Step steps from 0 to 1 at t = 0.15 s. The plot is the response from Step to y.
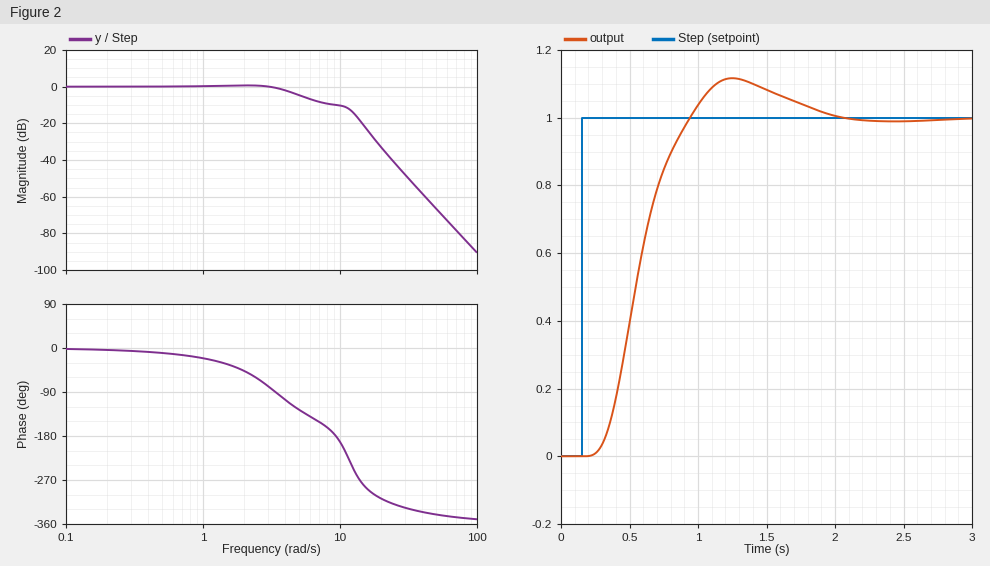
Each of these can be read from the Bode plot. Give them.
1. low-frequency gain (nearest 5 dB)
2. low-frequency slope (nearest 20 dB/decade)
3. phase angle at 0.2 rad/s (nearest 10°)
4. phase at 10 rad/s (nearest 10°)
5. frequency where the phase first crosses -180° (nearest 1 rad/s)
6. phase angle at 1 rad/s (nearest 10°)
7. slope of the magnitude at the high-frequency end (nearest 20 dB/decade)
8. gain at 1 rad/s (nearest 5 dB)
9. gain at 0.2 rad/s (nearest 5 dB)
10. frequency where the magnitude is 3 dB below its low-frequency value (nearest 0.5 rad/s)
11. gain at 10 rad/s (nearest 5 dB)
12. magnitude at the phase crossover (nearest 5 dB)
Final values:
0 dB
0 dB/decade
0°
-190°
9 rad/s
-20°
-80 dB/decade
0 dB
0 dB
4.5 rad/s
-10 dB
-10 dB
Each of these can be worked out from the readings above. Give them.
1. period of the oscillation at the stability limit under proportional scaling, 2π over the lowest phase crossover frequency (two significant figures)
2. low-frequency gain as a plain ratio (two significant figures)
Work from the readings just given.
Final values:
0.70 s
1.0
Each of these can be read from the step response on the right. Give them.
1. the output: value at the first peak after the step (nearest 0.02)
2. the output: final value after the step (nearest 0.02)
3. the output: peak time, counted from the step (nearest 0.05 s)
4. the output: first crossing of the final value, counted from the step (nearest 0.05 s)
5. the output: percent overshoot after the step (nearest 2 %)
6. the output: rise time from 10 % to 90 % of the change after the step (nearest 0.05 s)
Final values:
1.12
1.00
1.10 s
0.80 s
12 %
0.45 s
